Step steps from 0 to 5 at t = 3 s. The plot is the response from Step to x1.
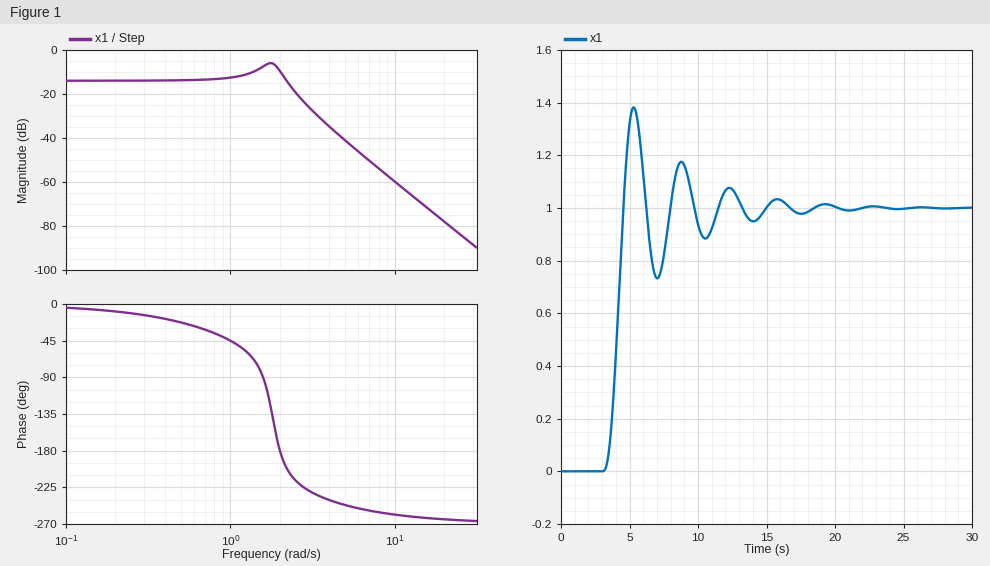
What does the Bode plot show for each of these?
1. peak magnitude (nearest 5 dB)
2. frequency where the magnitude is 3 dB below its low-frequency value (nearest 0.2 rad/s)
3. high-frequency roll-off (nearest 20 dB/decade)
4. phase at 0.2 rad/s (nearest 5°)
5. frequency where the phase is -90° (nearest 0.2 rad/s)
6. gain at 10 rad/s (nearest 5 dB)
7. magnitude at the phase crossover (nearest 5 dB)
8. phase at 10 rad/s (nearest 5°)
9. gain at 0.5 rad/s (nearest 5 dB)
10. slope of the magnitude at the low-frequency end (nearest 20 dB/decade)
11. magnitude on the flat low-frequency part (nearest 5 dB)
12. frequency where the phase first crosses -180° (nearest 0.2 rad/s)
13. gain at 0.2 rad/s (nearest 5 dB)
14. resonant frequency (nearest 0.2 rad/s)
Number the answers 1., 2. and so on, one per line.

1. -5 dB
2. 2.4 rad/s
3. -60 dB/decade
4. -10°
5. 1.6 rad/s
6. -60 dB
7. -10 dB
8. -260°
9. -15 dB
10. 0 dB/decade
11. -15 dB
12. 2.0 rad/s
13. -15 dB
14. 1.8 rad/s
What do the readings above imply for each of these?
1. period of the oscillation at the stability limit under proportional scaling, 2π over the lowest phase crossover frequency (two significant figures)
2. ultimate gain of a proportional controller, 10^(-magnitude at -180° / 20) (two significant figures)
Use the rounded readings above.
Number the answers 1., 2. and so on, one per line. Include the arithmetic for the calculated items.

1. 2π / 2 = 3.1 s
2. 10^(10 / 20) = 3.2
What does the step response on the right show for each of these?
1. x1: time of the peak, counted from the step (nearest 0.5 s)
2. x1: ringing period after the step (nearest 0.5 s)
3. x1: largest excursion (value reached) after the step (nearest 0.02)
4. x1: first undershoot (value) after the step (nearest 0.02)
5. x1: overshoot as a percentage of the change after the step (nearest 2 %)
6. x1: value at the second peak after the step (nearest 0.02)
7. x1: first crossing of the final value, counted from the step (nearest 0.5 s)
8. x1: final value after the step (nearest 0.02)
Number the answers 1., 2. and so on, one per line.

1. 2.5 s
2. 3.5 s
3. 1.38
4. 0.74
5. 38 %
6. 1.18
7. 1.5 s
8. 1.00
